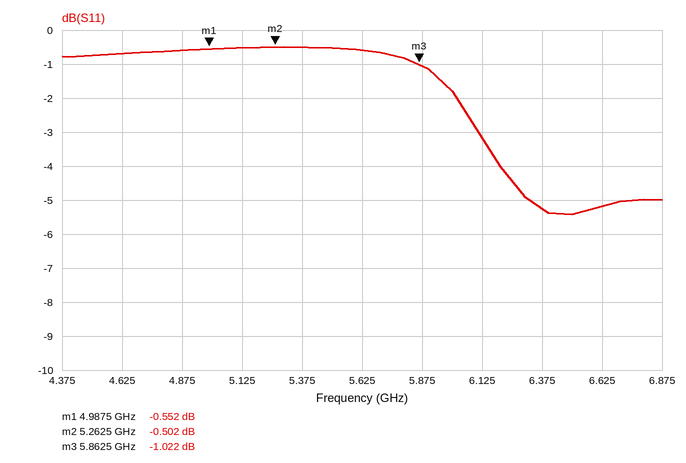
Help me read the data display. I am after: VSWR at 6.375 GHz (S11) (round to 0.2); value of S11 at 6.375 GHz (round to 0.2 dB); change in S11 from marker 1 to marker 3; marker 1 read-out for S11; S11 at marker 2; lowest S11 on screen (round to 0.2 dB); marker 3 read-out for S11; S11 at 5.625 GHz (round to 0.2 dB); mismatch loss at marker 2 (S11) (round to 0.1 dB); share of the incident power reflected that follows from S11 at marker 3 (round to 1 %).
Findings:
3.4
-5.2 dB
-0.470 dB
-0.552 dB
-0.502 dB
-5.4 dB
-1.022 dB
-0.6 dB
9.6 dB
79 %
